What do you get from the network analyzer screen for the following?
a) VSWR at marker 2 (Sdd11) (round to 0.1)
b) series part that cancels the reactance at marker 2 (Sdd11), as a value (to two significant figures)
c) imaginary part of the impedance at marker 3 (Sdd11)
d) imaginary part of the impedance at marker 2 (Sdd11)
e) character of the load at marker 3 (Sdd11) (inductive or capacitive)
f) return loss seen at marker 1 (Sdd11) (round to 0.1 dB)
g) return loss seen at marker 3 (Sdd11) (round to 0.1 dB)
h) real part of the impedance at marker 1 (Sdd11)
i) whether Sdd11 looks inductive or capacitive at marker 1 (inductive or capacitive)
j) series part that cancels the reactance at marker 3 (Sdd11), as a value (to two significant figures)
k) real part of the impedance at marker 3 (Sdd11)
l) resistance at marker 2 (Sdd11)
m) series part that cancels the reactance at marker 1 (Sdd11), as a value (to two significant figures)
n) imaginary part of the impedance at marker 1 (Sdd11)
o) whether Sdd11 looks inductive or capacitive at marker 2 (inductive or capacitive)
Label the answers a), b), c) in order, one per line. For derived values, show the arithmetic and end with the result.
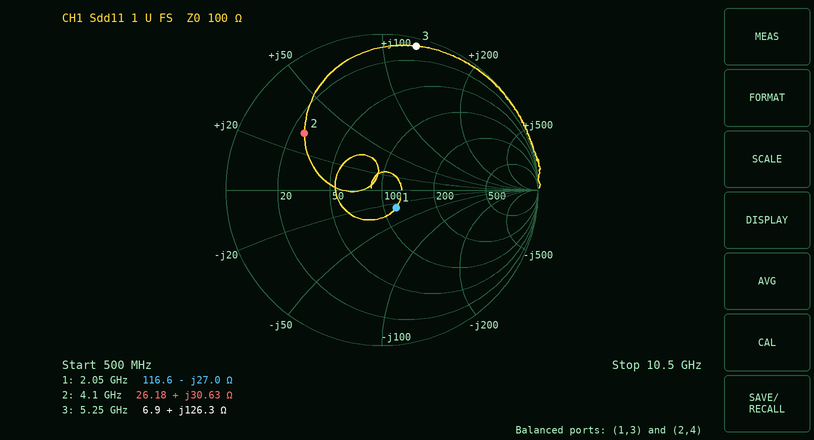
a) 4.2
b) C = 1/(2π × 4.1 GHz × 30.63 Ω) ≈ 1.3 pF
c) +126.3 Ω
d) +30.63 Ω
e) inductive
f) 16.8 dB
g) 0.5 dB
h) 116.6 Ω
i) capacitive
j) C = 1/(2π × 5.25 GHz × 126.3 Ω) ≈ 240 fF
k) 6.9 Ω
l) 26.18 Ω
m) L = 27 Ω/(2π × 2.05 GHz) ≈ 2.1 nH
n) -27.0 Ω
o) inductive
